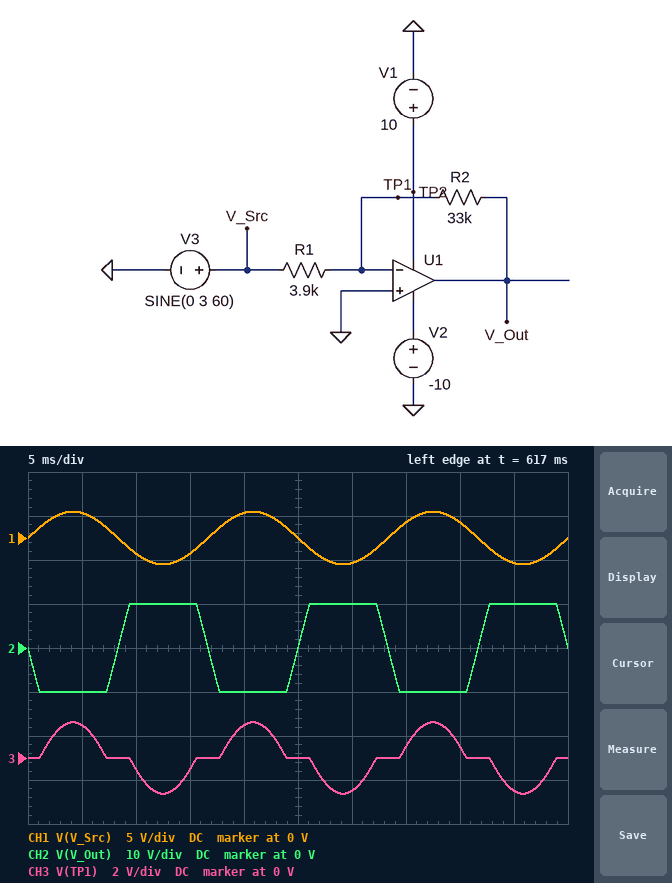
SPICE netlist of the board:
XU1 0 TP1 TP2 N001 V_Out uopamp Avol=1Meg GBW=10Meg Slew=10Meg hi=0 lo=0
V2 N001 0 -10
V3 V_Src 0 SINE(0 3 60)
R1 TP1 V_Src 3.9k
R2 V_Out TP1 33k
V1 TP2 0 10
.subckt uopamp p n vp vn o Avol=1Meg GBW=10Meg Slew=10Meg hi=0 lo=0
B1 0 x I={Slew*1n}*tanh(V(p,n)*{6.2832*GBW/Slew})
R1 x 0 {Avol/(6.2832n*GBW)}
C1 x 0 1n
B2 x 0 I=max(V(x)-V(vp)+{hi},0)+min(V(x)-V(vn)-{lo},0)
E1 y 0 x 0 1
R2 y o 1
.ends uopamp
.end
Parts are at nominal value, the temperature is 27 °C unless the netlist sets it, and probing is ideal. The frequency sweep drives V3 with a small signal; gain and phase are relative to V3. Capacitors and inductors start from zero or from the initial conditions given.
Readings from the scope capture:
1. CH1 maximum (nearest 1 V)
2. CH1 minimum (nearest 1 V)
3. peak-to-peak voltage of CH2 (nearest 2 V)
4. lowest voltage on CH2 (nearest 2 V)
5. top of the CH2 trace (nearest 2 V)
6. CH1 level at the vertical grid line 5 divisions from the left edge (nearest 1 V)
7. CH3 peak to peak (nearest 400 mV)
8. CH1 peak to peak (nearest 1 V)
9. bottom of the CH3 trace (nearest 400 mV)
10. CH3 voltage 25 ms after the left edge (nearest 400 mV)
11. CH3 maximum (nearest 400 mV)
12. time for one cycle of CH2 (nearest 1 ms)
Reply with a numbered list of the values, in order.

1. 3 V
2. -3 V
3. 20 V
4. -10 V
5. 10 V
6. 0 V
7. 3.2 V
8. 6 V
9. -1.6 V
10. 0 V
11. 1.6 V
12. 17 ms
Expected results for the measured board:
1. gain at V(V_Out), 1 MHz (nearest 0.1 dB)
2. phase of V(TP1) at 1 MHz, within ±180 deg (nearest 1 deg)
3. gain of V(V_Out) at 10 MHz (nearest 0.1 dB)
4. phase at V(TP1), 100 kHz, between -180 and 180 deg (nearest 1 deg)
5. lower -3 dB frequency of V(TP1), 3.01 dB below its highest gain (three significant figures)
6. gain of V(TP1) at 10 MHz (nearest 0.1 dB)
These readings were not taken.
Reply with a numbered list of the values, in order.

1. 15.8 dB
2. 47 deg
3. -1.0 dB
4. 85 deg
5. 1.06 MHz
6. -1.0 dB
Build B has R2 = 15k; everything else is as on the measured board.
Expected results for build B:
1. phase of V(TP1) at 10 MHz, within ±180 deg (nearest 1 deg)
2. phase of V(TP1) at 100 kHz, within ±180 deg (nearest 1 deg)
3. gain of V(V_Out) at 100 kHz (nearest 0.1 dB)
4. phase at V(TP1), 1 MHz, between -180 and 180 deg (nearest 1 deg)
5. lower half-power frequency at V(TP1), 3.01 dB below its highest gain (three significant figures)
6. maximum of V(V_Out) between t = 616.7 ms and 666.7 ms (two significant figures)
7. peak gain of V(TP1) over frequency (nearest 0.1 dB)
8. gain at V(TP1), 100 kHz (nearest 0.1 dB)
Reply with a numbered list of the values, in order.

1. 12 deg
2. 87 deg
3. 11.7 dB
4. 64 deg
5. 2.06 MHz
6. 10 V
7. -2.0 dB
8. -28.3 dB
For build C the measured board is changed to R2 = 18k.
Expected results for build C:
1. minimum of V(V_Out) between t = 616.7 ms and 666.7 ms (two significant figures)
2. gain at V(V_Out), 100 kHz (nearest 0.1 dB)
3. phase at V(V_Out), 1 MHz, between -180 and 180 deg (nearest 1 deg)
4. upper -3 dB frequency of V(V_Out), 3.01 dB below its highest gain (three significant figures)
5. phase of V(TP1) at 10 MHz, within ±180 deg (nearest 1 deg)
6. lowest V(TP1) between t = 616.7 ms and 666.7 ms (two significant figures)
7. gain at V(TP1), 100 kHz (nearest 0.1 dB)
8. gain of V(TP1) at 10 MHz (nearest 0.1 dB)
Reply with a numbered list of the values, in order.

1. -10 V
2. 13.3 dB
3. 151 deg
4. 1.78 MHz
5. 10 deg
6. -680 mV
7. -26.7 dB
8. -1.8 dB
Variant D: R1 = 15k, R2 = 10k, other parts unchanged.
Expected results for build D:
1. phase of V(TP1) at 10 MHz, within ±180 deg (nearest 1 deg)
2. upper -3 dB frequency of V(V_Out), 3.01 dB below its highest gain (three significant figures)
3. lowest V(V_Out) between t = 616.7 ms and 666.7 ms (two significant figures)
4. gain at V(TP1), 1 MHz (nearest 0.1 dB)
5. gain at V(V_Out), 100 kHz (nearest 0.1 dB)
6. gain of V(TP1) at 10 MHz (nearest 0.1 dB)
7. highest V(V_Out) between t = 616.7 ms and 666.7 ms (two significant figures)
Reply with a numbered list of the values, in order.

1. 31 deg
2. 6.00 MHz
3. -2.0 V
4. -23.6 dB
5. -3.5 dB
6. -9.3 dB
7. 2.0 V
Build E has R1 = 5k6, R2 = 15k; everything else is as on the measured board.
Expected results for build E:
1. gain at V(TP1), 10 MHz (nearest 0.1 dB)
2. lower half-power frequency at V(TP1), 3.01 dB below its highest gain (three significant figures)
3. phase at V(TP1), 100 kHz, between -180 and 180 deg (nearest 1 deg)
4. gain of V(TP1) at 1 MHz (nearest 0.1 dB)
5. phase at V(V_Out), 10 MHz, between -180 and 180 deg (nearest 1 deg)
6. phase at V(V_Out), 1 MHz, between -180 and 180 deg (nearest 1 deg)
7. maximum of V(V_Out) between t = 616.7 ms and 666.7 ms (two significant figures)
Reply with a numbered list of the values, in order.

1. -3.1 dB
2. 2.72 MHz
3. 88 deg
4. -12.0 dB
5. 105 deg
6. 160 deg
7. 8.0 V
